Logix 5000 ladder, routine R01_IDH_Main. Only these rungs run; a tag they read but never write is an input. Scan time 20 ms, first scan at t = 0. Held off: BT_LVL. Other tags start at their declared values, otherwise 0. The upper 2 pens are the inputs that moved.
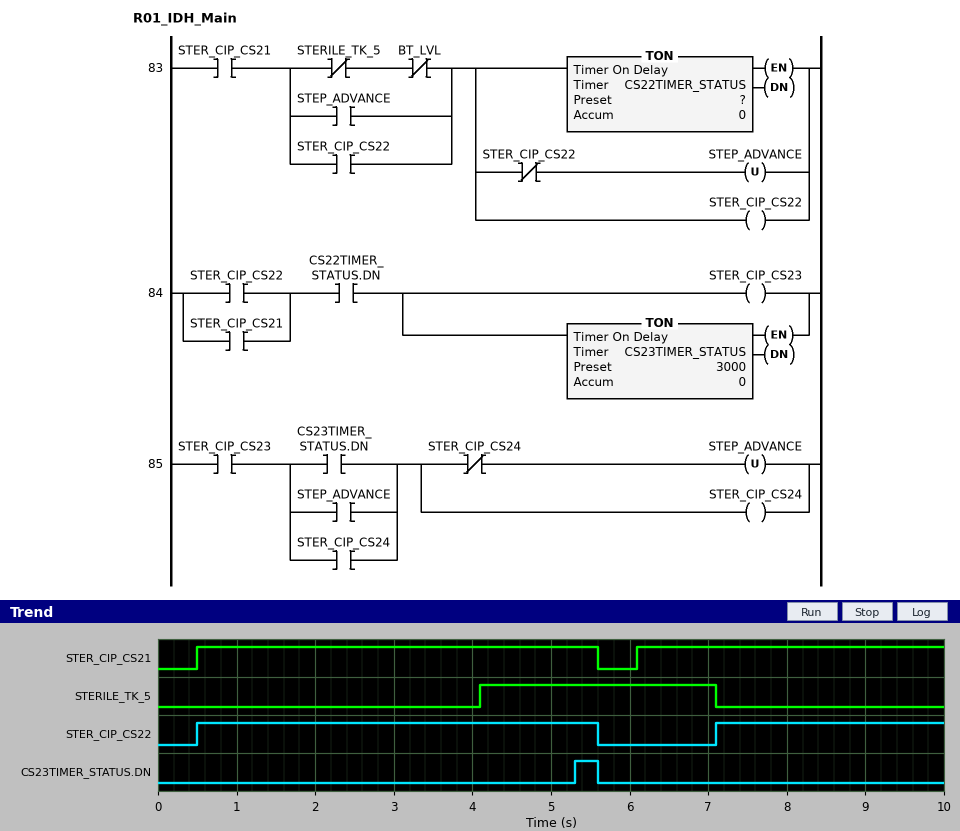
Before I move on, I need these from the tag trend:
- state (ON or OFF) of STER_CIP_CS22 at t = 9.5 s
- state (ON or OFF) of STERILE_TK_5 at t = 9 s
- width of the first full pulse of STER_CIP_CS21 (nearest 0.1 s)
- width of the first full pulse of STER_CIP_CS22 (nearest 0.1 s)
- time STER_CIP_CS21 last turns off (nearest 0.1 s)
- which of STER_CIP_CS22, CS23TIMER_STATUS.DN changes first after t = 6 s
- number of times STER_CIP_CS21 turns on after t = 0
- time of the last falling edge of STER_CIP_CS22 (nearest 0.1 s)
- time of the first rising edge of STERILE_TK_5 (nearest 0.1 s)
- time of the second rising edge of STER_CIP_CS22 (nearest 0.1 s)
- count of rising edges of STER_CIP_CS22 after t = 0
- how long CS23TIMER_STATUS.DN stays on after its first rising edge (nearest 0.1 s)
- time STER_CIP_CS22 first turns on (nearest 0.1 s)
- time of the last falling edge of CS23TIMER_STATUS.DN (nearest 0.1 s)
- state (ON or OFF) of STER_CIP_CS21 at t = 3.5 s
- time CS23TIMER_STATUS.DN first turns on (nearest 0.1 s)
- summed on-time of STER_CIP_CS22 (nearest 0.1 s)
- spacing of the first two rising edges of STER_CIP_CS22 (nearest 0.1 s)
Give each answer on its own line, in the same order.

ON
OFF
5.1 s
5.1 s
5.6 s
STER_CIP_CS22
2
5.6 s
4.1 s
7.1 s
2
0.3 s
0.5 s
5.6 s
ON
5.3 s
8.0 s
6.6 s
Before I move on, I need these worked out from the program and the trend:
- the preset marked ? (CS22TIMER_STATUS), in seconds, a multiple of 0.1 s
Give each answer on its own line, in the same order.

1.8 s
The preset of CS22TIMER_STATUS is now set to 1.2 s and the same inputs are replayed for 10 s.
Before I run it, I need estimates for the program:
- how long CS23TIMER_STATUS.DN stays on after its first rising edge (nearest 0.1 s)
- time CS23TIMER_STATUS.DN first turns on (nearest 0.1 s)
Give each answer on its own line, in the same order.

0.9 s
4.7 s
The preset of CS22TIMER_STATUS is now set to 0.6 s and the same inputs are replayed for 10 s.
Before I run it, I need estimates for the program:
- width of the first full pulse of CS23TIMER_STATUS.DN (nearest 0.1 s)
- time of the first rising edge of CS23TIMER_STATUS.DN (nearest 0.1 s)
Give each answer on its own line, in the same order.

1.5 s
4.1 s
